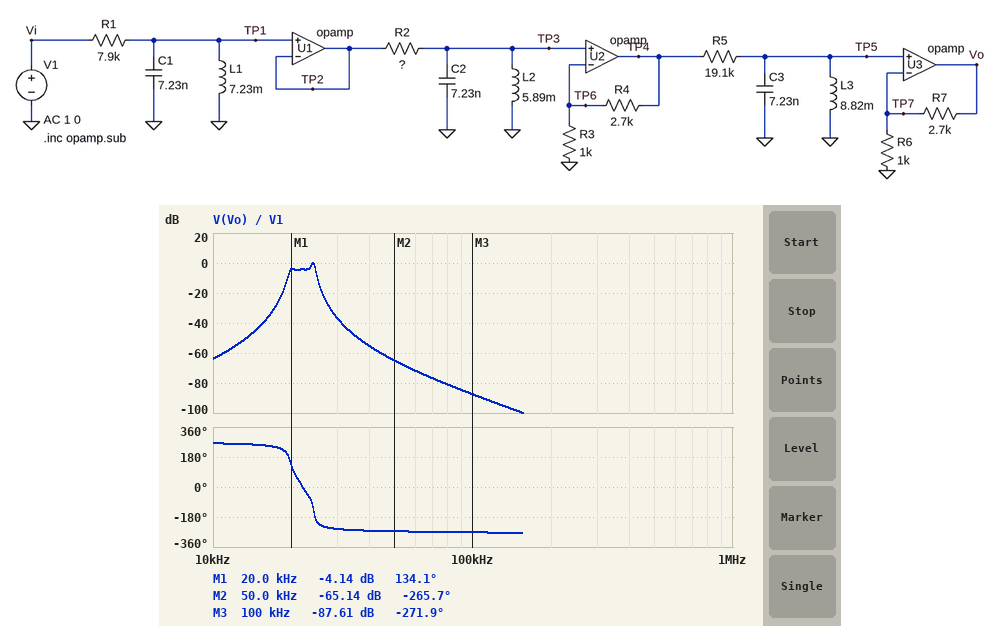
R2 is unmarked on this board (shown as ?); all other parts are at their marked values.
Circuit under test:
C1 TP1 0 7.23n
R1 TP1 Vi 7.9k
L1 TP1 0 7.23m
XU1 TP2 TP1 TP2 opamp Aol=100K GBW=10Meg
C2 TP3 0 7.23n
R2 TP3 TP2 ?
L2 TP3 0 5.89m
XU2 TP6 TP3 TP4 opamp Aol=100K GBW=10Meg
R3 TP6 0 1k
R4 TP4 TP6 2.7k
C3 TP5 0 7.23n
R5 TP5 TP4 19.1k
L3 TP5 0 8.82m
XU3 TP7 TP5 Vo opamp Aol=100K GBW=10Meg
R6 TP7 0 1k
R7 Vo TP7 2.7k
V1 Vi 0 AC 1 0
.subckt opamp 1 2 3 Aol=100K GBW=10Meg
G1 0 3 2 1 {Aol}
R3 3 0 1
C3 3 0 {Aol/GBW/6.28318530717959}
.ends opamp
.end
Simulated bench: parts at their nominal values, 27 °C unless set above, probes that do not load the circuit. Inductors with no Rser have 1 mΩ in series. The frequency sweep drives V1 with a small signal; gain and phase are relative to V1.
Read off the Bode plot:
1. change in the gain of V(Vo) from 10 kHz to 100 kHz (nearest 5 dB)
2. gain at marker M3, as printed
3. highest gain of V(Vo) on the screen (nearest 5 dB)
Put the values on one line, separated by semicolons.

-25 dB; -87.61 dB; 0 dB
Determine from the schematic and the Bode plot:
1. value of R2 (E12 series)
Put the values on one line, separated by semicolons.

27 kΩ
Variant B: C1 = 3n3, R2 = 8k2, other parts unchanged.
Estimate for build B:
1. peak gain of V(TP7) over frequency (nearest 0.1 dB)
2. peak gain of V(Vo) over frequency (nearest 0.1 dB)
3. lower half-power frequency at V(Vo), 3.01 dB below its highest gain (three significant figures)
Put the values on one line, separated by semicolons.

-15.0 dB; -3.6 dB; 19.5 kHz
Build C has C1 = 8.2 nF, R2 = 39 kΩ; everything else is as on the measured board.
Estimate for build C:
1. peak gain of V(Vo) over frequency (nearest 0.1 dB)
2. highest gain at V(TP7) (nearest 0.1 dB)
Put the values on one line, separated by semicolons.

-3.0 dB; -14.4 dB
